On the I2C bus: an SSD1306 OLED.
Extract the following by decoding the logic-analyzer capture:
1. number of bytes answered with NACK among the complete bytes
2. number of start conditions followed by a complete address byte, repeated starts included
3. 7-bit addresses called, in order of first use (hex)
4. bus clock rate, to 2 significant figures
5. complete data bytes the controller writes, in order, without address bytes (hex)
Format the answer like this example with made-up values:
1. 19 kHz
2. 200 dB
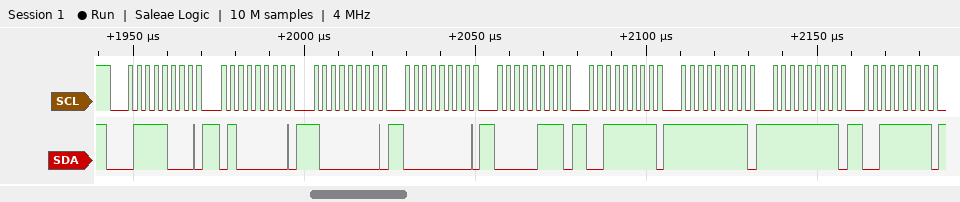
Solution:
1. 0
2. 1
3. 0x3C
4. 400 kHz
5. 40 80 00 07 3F FF FF 3F
